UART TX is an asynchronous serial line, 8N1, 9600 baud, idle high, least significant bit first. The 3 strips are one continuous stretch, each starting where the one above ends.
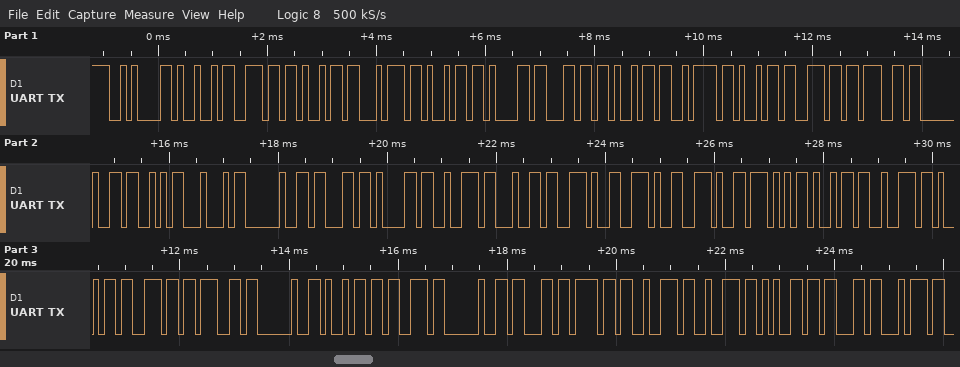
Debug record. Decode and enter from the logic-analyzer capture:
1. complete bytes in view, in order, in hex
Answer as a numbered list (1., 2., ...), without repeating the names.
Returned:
1. 0x0A 0x49 0x6E 0x69 0x74 0x69 0x61 0x6C 0x69 0x7A 0x69 0x6E 0x67 0x20 0x53 0x44 0x20 0x63 0x61 0x72 0x64 0x2E 0x2E 0x2E 0x57 0x69 0x72 0x69 0x6E 0x67 0x20 0x69 0x73 0x20 0x63 0x6F 0x72 0x72 0x65 0x63 0x74
